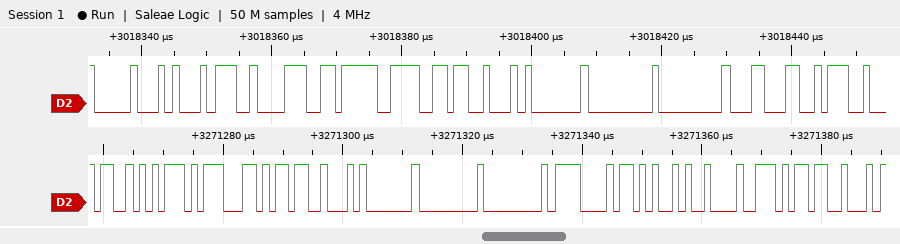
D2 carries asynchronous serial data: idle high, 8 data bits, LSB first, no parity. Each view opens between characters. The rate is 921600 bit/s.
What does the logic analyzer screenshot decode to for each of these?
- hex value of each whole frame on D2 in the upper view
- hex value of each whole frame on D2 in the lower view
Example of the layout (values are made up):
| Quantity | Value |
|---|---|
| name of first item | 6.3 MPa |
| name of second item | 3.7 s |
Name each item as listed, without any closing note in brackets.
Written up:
| Quantity | Value |
|---|---|
| hex value of each whole frame on D2 in the upper view | 10, D1, C2, F6, 9E, 13, 01, 00, 00, 8C, 3A |
| hex value of each whole frame on D2 in the lower view | 53, D7, AC, 13, 01, 00, 00, 0F, 2B, 09, AE, 13 |
